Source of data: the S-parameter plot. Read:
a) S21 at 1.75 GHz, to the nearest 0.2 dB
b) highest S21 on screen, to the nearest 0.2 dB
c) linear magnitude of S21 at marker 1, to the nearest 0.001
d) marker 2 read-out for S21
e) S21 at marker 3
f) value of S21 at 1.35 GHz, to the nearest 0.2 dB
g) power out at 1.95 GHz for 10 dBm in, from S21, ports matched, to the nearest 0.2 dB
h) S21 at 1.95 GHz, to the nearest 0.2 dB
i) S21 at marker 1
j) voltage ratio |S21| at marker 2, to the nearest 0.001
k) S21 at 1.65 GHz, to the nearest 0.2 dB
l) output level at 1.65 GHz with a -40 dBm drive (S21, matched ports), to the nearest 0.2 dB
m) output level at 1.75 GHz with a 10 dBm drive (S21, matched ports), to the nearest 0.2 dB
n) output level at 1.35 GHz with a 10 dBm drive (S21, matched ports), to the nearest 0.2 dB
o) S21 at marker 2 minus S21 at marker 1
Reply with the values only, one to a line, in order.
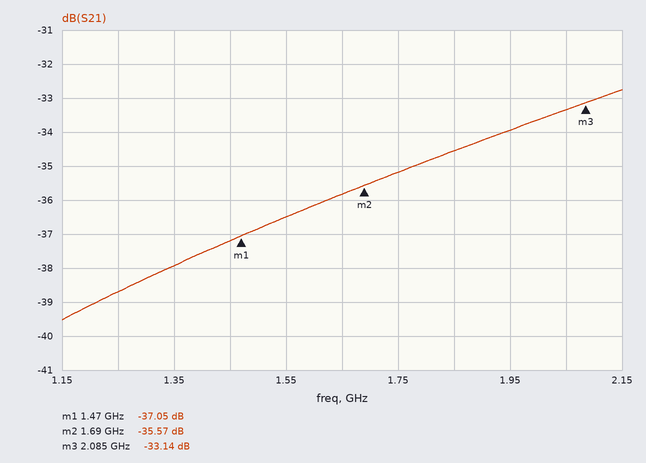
-35.2 dB
-32.8 dB
0.014
-35.57 dB
-33.14 dB
-38.0 dB
-24.0 dBm
-34.0 dB
-37.05 dB
0.017
-35.8 dB
-75.8 dBm
-25.2 dBm
-28.0 dBm
1.48 dB
